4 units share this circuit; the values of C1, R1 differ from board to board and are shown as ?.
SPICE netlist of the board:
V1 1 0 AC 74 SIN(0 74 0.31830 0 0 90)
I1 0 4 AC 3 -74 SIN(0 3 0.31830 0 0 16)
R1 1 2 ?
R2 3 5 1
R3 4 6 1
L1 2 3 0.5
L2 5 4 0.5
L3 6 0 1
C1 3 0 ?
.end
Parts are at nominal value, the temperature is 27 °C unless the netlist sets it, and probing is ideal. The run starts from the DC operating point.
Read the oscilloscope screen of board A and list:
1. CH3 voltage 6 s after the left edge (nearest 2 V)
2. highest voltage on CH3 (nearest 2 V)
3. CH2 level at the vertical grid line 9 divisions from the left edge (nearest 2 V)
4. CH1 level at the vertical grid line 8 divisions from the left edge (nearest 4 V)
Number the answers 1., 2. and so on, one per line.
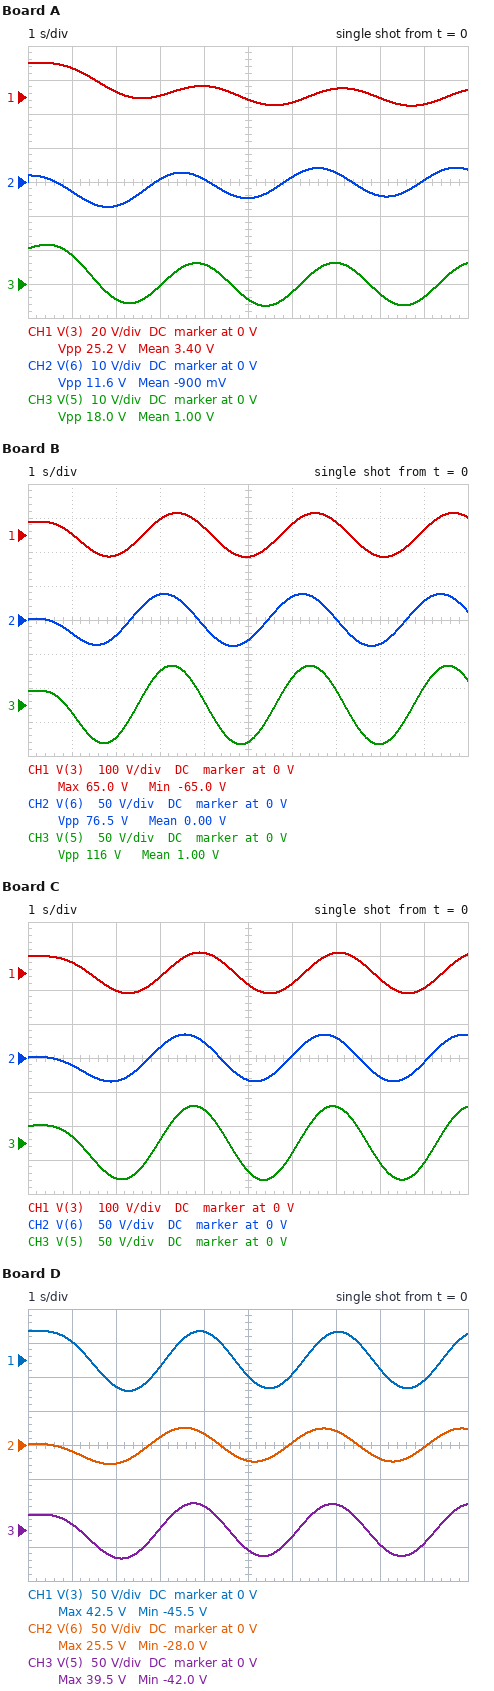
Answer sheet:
1. -2 V
2. 12 V
3. 0 V
4. 0 V
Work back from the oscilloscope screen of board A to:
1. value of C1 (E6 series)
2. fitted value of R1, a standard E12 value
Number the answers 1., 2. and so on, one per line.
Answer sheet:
1. 1.5 F
2. 5.6 Ω
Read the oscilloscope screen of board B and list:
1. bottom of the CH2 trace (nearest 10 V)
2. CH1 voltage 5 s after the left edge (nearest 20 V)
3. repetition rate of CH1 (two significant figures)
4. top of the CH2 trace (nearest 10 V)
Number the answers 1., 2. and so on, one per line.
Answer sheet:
1. -40 V
2. -60 V
3. 320 mHz
4. 40 V
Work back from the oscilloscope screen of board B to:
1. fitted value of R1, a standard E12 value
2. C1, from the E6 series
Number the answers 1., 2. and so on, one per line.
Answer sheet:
1. 1.8 Ω
2. 220 mF
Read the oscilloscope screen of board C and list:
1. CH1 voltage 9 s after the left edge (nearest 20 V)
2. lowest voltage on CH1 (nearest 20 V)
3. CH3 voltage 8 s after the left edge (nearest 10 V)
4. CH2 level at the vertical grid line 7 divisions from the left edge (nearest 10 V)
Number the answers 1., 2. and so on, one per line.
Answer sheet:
1. -40 V
2. -60 V
3. -30 V
4. 30 V
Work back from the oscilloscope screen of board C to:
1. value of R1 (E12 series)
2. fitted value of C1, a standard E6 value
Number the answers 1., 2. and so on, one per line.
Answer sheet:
1. 1 Ω
2. 680 mF
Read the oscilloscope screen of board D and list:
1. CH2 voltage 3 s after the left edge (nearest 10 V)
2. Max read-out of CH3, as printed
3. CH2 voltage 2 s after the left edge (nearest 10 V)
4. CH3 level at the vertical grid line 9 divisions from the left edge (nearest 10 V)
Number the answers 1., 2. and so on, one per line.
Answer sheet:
1. 10 V
2. 39.5 V
3. -30 V
4. -20 V
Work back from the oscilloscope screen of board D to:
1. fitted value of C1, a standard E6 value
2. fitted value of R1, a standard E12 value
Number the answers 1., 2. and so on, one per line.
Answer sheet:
1. 680 mF
2. 1.5 Ω
